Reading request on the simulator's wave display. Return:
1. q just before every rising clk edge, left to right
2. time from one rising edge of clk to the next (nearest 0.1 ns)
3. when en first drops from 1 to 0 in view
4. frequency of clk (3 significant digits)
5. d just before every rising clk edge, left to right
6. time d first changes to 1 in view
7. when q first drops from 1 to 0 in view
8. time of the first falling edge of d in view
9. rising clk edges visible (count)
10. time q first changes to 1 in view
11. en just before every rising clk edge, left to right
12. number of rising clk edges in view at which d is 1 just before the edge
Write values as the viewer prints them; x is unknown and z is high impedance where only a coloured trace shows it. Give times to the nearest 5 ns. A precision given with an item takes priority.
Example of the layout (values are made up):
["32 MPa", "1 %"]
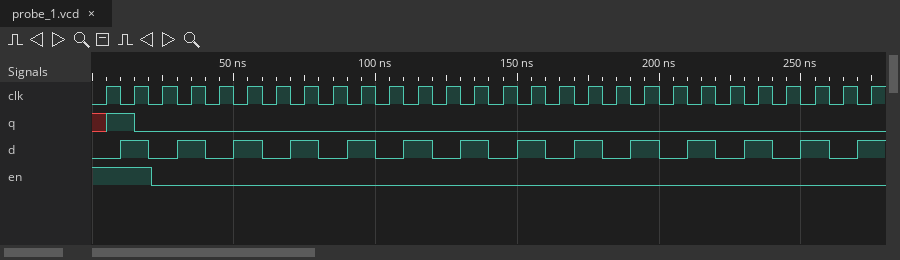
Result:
["x 1 0 0 0 0 0 0 0 0 0 0 0 0 0 0 0 0 0 0 0 0 0 0 0 0 0 0", "10 ns", "20 ns", "100 MHz", "0 1 0 1 0 1 0 1 0 1 0 1 0 1 0 1 0 1 0 1 0 1 0 1 0 1 0 1", "10 ns", "15 ns", "20 ns", "28", "5 ns", "1 1 0 0 0 0 0 0 0 0 0 0 0 0 0 0 0 0 0 0 0 0 0 0 0 0 0 0", "14"]
